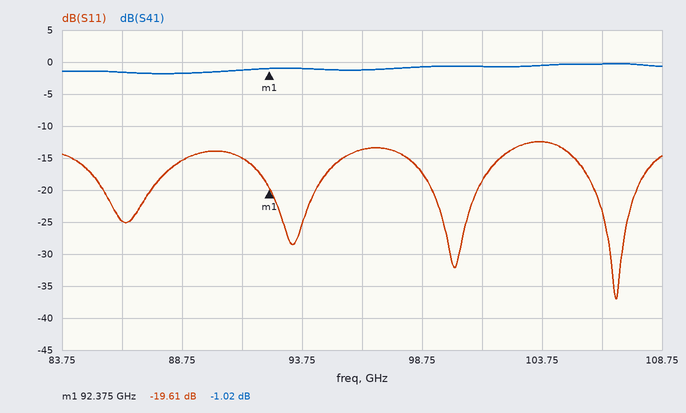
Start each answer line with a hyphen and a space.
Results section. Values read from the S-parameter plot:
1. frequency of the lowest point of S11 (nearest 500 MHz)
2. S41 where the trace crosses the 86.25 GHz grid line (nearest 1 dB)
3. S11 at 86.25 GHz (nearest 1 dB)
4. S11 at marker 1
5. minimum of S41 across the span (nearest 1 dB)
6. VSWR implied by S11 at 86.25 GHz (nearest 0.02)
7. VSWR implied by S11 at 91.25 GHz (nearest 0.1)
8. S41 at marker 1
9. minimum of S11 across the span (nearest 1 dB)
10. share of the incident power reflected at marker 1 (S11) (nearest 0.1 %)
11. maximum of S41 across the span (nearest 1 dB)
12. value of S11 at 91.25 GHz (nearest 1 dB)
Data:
- 107.0 GHz
- -2 dB
- -25 dB
- -19.61 dB
- -2 dB
- 1.12
- 1.4
- -1.02 dB
- -37 dB
- 1.1 %
- 0 dB
- -15 dB
